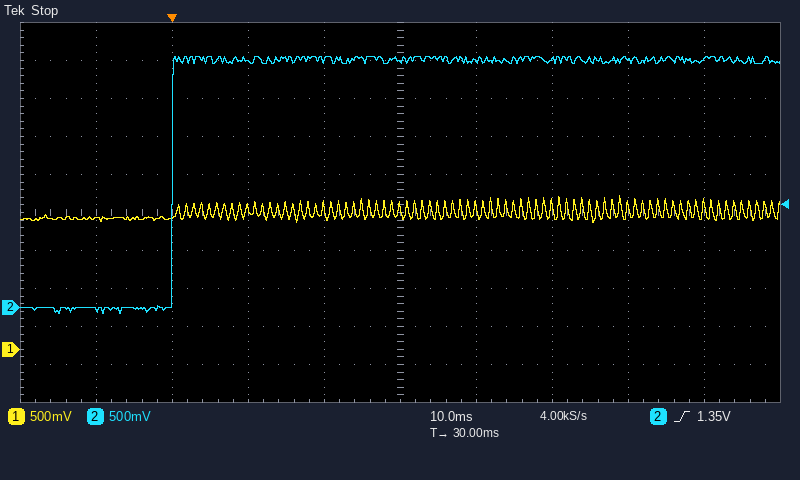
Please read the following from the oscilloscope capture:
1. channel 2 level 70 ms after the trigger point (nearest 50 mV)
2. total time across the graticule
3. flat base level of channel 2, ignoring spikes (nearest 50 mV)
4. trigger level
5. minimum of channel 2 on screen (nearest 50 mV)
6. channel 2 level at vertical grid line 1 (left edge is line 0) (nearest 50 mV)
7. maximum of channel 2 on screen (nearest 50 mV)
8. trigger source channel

3.25 V
100 ms
0 mV
1.35 V
-100 mV
-50 mV
3.30 V
channel 2
